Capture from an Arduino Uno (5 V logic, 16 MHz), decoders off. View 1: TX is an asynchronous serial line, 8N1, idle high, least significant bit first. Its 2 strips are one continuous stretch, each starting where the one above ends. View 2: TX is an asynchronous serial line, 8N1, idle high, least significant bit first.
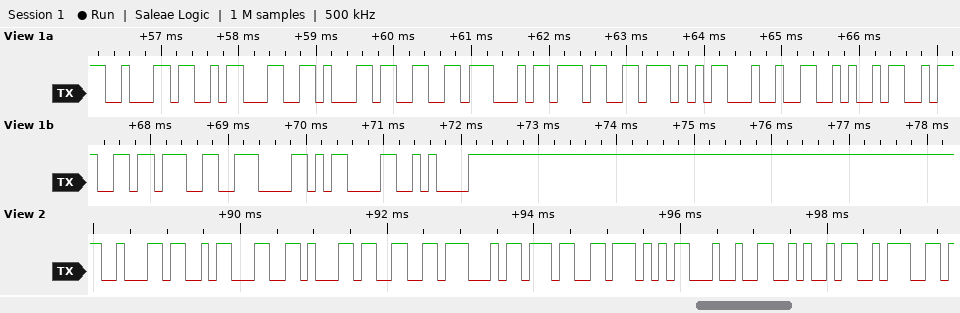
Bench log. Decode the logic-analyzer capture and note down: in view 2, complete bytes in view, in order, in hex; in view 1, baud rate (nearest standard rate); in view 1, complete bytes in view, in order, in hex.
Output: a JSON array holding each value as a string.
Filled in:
["62 1A 16 33 47 37 57 24 4A 3A", "9600 baud", "62 1A 16 33 47 37 57 24 4A 3A 3B 0E 0D 0A"]
